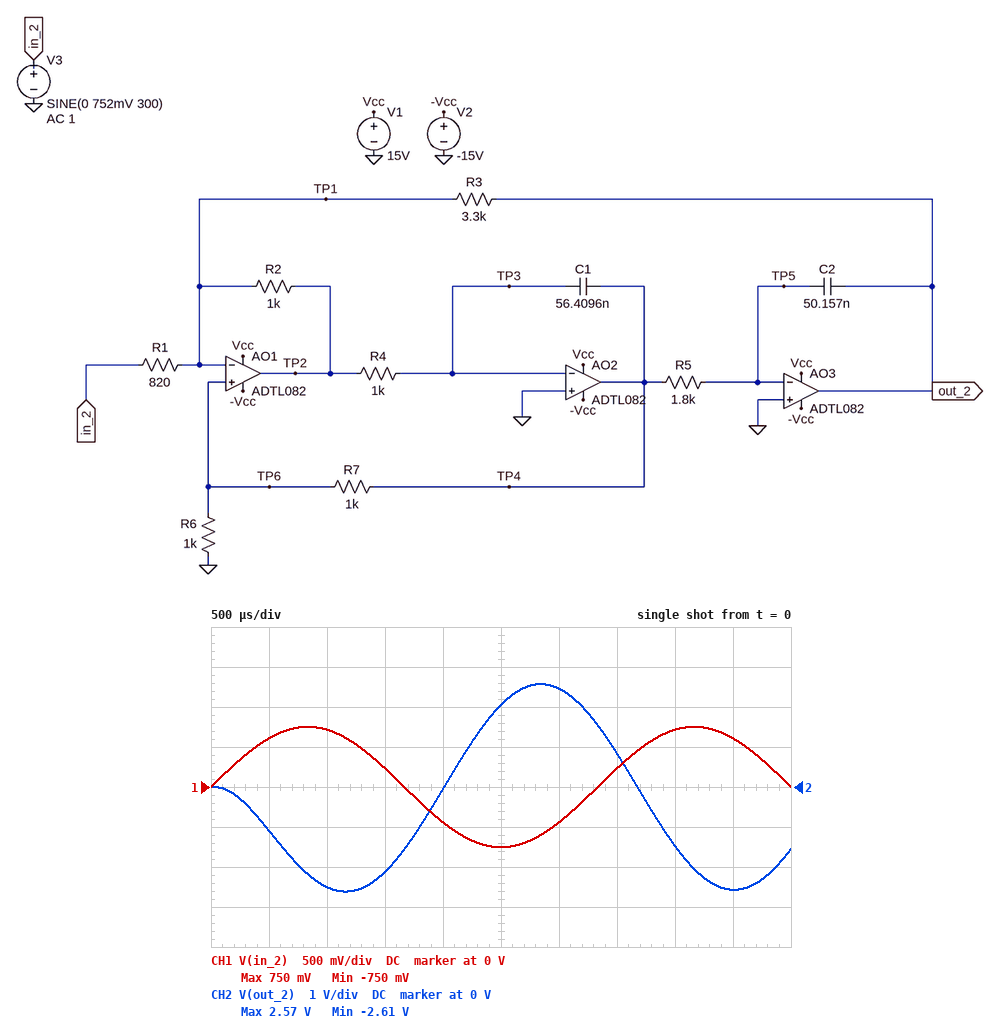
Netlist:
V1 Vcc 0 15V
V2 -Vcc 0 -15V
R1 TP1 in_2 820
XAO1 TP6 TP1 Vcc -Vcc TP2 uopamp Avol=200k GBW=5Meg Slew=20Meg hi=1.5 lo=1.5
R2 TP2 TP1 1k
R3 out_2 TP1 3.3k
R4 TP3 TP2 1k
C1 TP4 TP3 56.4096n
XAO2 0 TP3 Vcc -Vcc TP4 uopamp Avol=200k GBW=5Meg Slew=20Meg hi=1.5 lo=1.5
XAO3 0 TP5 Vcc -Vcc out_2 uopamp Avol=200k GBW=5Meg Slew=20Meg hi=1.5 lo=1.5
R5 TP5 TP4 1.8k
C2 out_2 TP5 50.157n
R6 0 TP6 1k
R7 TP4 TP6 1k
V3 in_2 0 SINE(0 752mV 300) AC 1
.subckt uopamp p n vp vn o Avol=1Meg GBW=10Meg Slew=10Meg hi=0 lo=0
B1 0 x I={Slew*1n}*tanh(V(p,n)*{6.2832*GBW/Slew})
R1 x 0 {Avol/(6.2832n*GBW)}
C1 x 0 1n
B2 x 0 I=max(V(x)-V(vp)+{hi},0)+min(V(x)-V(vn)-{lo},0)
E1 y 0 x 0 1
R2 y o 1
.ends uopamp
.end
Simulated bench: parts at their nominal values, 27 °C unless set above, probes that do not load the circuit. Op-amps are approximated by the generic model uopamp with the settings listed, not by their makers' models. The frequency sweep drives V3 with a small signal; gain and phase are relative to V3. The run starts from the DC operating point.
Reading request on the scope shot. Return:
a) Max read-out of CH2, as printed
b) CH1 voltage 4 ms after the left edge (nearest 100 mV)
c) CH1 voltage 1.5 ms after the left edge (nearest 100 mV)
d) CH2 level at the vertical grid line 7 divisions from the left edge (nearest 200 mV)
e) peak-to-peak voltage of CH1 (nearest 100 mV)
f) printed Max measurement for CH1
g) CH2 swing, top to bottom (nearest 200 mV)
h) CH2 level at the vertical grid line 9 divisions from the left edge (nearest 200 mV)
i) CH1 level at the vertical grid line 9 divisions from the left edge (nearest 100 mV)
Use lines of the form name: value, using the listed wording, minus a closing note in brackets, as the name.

Max read-out of CH2, as printed: 2.57 V
CH1 voltage 4 ms after the left edge: 700 mV
CH1 voltage 1.5 ms after the left edge: 200 mV
CH2 level at the vertical grid line 7 divisions from the left edge: 800 mV
peak-to-peak voltage of CH1: 1.5 V
printed Max measurement for CH1: 750 mV
CH2 swing, top to bottom: 5.2 V
CH2 level at the vertical grid line 9 divisions from the left edge: -2.6 V
CH1 level at the vertical grid line 9 divisions from the left edge: 600 mV
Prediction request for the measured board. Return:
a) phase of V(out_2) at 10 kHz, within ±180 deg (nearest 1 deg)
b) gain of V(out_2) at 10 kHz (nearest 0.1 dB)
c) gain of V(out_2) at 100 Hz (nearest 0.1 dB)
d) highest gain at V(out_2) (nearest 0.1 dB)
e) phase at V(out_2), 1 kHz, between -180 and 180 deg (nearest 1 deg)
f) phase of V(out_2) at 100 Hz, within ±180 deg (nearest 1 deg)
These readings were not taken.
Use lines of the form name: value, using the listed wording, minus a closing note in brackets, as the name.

phase of V(out_2) at 10 kHz, within ±180 deg: 19 deg
gain of V(out_2) at 10 kHz: -24.7 dB
gain of V(out_2) at 100 Hz: 11.9 dB
highest gain at V(out_2): 12.1 dB
phase at V(out_2), 1 kHz, between -180 and 180 deg: 98 deg
phase of V(out_2) at 100 Hz, within ±180 deg: 167 deg
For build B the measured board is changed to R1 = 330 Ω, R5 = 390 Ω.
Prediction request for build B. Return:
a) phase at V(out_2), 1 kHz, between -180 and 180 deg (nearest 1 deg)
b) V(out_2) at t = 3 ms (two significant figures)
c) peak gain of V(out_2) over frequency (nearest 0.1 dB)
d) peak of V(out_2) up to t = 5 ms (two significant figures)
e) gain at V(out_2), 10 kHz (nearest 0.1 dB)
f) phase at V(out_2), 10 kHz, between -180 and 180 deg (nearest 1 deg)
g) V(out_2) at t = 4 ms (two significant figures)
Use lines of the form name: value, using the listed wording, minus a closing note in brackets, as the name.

phase at V(out_2), 1 kHz, between -180 and 180 deg: 134 deg
V(out_2) at t = 3 ms: 5.7 V
peak gain of V(out_2) over frequency: 20.0 dB
peak of V(out_2) up to t = 5 ms: 7.4 V
gain at V(out_2), 10 kHz: -4.1 dB
phase at V(out_2), 10 kHz, between -180 and 180 deg: 33 deg
V(out_2) at t = 4 ms: -6.2 V
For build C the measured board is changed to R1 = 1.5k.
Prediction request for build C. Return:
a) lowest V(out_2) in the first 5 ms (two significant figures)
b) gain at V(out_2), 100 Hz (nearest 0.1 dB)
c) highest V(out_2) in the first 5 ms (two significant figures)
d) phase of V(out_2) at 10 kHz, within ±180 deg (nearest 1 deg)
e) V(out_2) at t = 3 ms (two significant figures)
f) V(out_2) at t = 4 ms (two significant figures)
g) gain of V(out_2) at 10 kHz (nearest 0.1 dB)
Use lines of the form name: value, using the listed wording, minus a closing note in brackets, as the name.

lowest V(out_2) in the first 5 ms: -1.5 V
gain at V(out_2), 100 Hz: 6.8 dB
highest V(out_2) in the first 5 ms: 1.5 V
phase of V(out_2) at 10 kHz, within ±180 deg: 15 deg
V(out_2) at t = 3 ms: 1.4 V
V(out_2) at t = 4 ms: -1.0 V
gain of V(out_2) at 10 kHz: -29.8 dB
